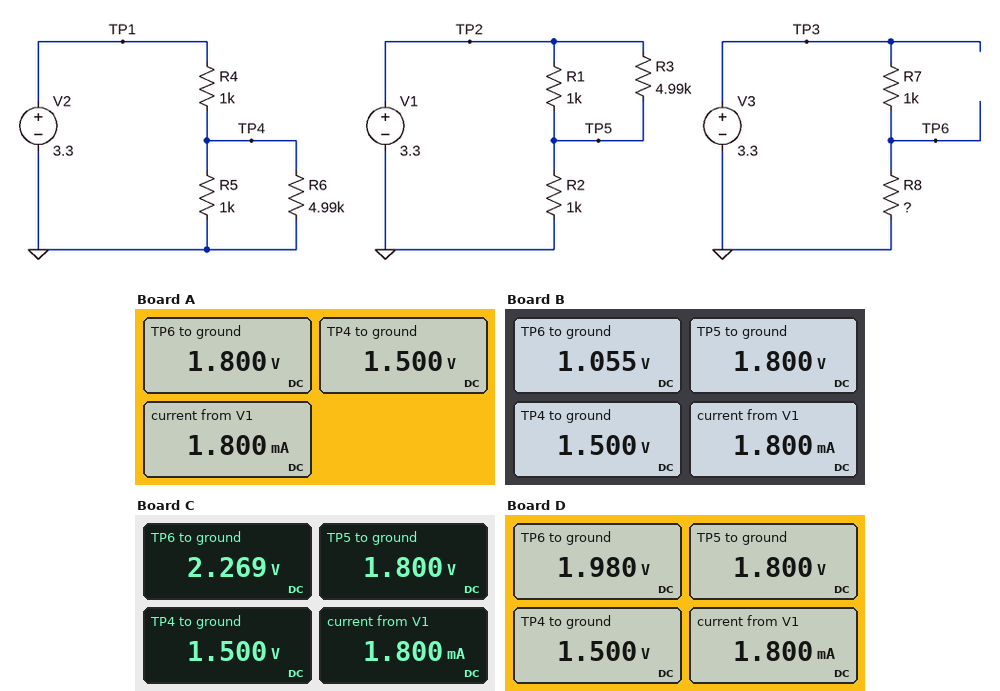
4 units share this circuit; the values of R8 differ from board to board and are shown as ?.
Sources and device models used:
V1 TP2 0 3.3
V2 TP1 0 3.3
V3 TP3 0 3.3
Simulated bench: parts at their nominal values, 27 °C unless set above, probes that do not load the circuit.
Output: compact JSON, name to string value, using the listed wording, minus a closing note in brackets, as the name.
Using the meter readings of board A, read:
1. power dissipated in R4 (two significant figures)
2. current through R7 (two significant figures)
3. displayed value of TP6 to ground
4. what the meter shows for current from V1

{"power dissipated in R4": "3.2 mW", "current through R7": "1.5 mA", "displayed value of TP6 to ground": "1.800 V", "what the meter shows for current from V1": "1.800 mA"}
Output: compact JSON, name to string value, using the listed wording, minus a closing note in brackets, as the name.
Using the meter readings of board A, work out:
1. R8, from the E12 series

{"R8, from the E12 series": "1.2 kΩ"}
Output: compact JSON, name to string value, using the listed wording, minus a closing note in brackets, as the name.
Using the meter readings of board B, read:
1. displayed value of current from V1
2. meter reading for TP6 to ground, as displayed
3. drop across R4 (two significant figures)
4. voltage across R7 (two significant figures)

{"displayed value of current from V1": "1.800 mA", "meter reading for TP6 to ground, as displayed": "1.055 V", "drop across R4": "1.8 V", "voltage across R7": "2.2 V"}
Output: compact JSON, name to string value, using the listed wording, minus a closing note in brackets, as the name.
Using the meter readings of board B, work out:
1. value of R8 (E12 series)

{"value of R8": "470 Ω"}
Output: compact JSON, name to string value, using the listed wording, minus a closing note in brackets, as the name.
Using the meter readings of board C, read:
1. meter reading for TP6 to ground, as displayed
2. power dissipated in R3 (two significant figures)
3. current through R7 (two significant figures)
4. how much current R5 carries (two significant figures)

{"meter reading for TP6 to ground, as displayed": "2.269 V", "power dissipated in R3": "450 µW", "current through R7": "1.0 mA", "how much current R5 carries": "1.5 mA"}
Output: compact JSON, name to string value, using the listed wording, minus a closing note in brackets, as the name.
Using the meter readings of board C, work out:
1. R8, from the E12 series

{"R8, from the E12 series": "2.2 kΩ"}
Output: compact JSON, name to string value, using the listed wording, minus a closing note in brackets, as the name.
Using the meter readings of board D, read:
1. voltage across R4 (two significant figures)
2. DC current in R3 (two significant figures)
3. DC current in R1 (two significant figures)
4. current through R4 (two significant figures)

{"voltage across R4": "1.8 V", "DC current in R3": "300 µA", "DC current in R1": "1.5 mA", "current through R4": "1.8 mA"}
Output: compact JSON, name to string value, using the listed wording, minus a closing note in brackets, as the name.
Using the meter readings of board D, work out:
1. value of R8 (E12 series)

{"value of R8": "1.5 kΩ"}
